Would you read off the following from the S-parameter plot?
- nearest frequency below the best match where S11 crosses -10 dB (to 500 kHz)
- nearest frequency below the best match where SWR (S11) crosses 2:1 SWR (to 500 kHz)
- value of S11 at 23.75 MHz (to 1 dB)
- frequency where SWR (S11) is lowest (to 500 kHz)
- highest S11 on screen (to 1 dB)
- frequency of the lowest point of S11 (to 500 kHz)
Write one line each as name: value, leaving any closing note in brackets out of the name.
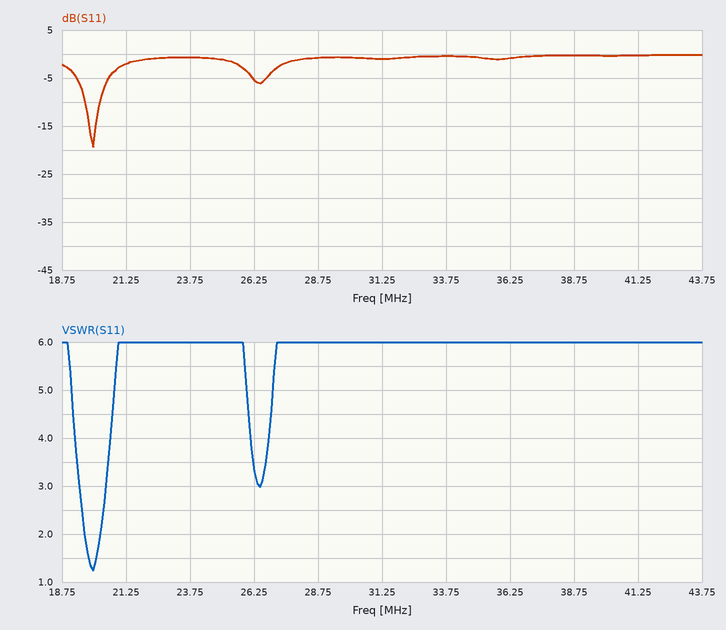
nearest frequency below the best match where S11 crosses -10 dB: 19.5 MHz
nearest frequency below the best match where SWR (S11) crosses 2:1 SWR: 19.5 MHz
value of S11 at 23.75 MHz: -1 dB
frequency where SWR (S11) is lowest: 20.0 MHz
highest S11 on screen: 0 dB
frequency of the lowest point of S11: 20.0 MHz
